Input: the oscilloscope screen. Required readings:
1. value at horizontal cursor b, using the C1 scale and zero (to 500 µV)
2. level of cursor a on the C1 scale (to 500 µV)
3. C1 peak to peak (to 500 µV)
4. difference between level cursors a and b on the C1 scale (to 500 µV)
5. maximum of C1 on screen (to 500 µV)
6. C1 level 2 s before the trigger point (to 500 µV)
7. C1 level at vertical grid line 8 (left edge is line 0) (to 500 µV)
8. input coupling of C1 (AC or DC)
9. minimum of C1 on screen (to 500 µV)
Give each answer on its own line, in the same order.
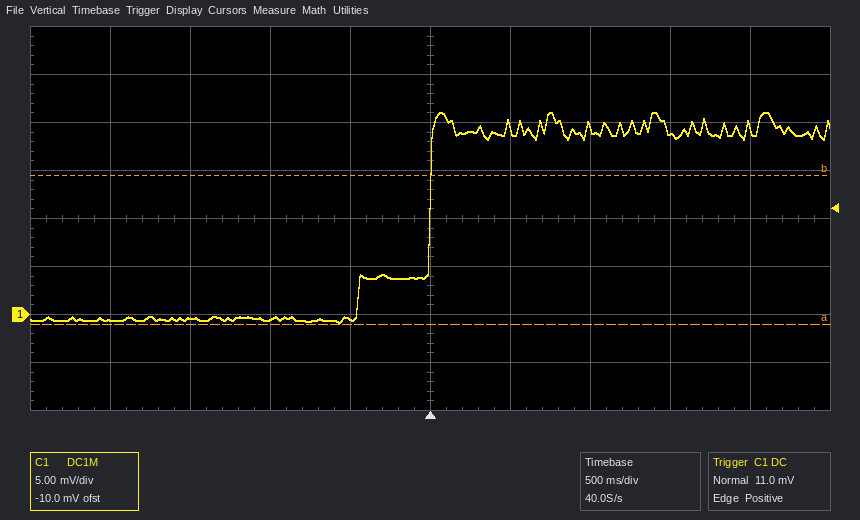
14.5 mV
-1.0 mV
22.0 mV
15.5 mV
21.0 mV
-500 µV
19.0 mV
DC
-1.0 mV
